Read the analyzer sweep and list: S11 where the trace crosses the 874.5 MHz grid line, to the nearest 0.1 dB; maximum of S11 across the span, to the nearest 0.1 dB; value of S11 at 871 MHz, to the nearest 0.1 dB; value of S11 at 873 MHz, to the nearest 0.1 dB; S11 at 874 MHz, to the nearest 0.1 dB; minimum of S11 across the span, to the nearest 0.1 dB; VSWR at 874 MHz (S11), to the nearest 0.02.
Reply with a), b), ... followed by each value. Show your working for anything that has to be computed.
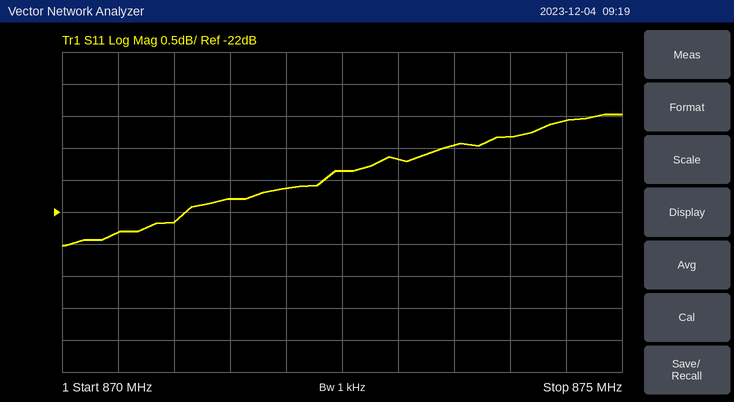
a) -20.6 dB
b) -20.5 dB
c) -22.2 dB
d) -21.2 dB
e) -20.8 dB
f) -22.5 dB
g) |Γ| = 10^(-20.8/20) = 0.0912; VSWR = (1 + 0.0912)/(1 − 0.0912) ≈ 1.20
